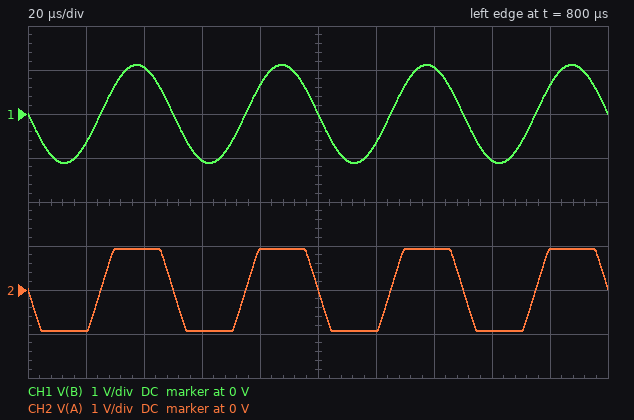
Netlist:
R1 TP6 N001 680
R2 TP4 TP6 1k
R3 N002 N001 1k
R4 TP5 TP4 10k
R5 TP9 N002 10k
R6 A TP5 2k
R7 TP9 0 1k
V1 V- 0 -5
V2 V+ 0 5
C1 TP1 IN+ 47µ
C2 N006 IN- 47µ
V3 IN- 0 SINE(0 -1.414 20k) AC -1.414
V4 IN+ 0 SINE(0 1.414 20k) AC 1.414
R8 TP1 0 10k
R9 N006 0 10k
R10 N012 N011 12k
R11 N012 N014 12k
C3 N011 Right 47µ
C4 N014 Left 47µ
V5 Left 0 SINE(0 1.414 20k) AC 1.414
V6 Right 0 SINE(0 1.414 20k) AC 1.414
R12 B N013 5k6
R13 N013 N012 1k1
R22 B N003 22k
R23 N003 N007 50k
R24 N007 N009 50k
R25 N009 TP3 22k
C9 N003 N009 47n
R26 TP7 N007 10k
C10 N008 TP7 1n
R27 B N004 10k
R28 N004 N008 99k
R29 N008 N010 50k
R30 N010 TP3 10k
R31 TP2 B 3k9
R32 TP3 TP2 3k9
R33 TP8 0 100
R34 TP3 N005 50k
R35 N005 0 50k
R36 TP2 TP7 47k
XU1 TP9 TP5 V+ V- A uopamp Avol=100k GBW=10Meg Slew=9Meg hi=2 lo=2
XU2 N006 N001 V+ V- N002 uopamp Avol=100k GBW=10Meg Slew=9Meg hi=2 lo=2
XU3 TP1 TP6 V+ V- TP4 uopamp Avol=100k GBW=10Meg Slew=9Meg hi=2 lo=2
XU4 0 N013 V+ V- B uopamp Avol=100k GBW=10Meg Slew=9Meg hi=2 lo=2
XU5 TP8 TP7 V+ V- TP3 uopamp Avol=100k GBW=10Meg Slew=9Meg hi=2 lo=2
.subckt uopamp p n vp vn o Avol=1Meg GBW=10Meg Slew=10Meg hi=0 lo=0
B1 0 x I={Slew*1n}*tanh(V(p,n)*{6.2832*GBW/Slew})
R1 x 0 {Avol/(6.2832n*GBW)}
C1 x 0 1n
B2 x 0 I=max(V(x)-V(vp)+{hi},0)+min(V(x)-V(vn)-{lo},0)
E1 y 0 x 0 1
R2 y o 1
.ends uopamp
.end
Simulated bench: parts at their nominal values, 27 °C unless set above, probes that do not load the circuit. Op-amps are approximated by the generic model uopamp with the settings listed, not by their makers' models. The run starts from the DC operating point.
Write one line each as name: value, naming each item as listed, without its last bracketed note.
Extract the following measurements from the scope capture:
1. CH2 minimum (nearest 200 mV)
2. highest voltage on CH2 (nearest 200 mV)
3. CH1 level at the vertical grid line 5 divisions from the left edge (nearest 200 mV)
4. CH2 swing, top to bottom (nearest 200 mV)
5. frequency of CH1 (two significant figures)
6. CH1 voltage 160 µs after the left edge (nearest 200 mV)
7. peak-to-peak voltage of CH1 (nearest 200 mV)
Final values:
CH2 minimum: -1.0 V
highest voltage on CH2: 1.0 V
CH1 level at the vertical grid line 5 divisions from the left edge: 0 V
CH2 swing, top to bottom: 1.8 V
frequency of CH1: 20 kHz
CH1 voltage 160 µs after the left edge: -1.0 V
peak-to-peak voltage of CH1: 2.2 V
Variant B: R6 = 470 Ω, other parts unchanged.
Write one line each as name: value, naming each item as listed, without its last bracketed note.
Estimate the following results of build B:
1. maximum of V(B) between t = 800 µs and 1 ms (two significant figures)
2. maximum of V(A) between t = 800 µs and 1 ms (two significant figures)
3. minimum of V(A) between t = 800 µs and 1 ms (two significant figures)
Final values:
maximum of V(B) between t = 800 µs and 1 ms: 1.1 V
maximum of V(A) between t = 800 µs and 1 ms: 430 mV
minimum of V(A) between t = 800 µs and 1 ms: -430 mV
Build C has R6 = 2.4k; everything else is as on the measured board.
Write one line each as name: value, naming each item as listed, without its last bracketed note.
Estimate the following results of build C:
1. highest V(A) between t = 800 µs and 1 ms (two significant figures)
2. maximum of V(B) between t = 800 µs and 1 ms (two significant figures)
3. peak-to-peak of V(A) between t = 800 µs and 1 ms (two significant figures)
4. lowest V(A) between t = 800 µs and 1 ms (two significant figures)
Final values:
highest V(A) between t = 800 µs and 1 ms: 1.1 V
maximum of V(B) between t = 800 µs and 1 ms: 1.1 V
peak-to-peak of V(A) between t = 800 µs and 1 ms: 2.1 V
lowest V(A) between t = 800 µs and 1 ms: -1.1 V
